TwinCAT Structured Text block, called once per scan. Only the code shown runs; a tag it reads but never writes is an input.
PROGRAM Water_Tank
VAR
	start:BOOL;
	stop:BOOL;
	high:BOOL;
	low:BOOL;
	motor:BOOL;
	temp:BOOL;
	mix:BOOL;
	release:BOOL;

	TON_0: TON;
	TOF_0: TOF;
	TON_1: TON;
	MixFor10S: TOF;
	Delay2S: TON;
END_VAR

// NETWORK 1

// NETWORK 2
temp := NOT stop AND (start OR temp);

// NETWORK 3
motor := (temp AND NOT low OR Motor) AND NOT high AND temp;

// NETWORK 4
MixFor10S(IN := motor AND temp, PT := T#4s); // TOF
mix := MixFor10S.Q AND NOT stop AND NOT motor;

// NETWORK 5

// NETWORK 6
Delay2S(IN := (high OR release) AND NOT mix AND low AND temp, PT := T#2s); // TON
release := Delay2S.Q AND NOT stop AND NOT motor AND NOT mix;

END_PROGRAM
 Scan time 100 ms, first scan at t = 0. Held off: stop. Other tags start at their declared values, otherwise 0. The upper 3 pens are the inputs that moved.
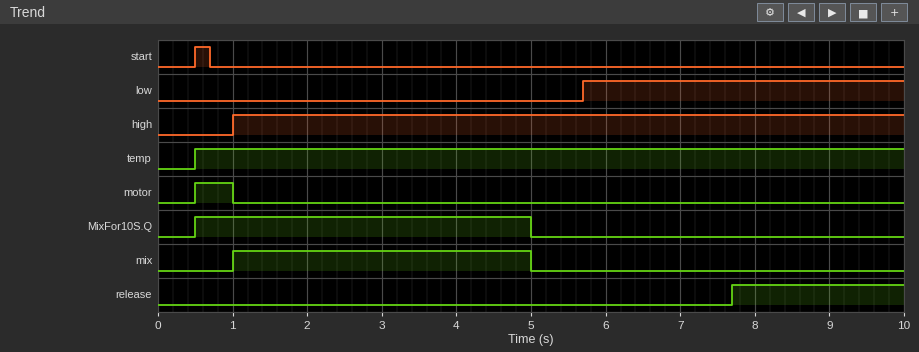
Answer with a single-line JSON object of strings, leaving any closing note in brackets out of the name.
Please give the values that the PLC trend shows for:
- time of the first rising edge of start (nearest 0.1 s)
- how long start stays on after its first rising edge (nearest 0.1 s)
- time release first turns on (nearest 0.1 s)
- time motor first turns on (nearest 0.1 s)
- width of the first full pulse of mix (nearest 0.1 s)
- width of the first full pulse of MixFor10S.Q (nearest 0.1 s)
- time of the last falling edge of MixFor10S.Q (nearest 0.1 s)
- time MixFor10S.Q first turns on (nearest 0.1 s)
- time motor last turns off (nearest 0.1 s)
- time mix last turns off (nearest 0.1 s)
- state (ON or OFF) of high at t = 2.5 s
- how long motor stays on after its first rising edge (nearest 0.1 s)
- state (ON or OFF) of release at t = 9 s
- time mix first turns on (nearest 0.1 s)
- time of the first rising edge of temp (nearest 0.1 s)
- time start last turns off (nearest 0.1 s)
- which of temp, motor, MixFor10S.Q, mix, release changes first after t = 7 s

{"time of the first rising edge of start": "0.5 s", "how long start stays on after its first rising edge": "0.2 s", "time release first turns on": "7.7 s", "time motor first turns on": "0.5 s", "width of the first full pulse of mix": "4.0 s", "width of the first full pulse of MixFor10S.Q": "4.5 s", "time of the last falling edge of MixFor10S.Q": "5.0 s", "time MixFor10S.Q first turns on": "0.5 s", "time motor last turns off": "1.0 s", "time mix last turns off": "5.0 s", "state (ON or OFF) of high at t = 2.5 s": "ON", "how long motor stays on after its first rising edge": "0.5 s", "state (ON or OFF) of release at t = 9 s": "ON", "time mix first turns on": "1.0 s", "time of the first rising edge of temp": "0.5 s", "time start last turns off": "0.7 s", "which of temp, motor, MixFor10S.Q, mix, release changes first after t = 7 s": "release"}
